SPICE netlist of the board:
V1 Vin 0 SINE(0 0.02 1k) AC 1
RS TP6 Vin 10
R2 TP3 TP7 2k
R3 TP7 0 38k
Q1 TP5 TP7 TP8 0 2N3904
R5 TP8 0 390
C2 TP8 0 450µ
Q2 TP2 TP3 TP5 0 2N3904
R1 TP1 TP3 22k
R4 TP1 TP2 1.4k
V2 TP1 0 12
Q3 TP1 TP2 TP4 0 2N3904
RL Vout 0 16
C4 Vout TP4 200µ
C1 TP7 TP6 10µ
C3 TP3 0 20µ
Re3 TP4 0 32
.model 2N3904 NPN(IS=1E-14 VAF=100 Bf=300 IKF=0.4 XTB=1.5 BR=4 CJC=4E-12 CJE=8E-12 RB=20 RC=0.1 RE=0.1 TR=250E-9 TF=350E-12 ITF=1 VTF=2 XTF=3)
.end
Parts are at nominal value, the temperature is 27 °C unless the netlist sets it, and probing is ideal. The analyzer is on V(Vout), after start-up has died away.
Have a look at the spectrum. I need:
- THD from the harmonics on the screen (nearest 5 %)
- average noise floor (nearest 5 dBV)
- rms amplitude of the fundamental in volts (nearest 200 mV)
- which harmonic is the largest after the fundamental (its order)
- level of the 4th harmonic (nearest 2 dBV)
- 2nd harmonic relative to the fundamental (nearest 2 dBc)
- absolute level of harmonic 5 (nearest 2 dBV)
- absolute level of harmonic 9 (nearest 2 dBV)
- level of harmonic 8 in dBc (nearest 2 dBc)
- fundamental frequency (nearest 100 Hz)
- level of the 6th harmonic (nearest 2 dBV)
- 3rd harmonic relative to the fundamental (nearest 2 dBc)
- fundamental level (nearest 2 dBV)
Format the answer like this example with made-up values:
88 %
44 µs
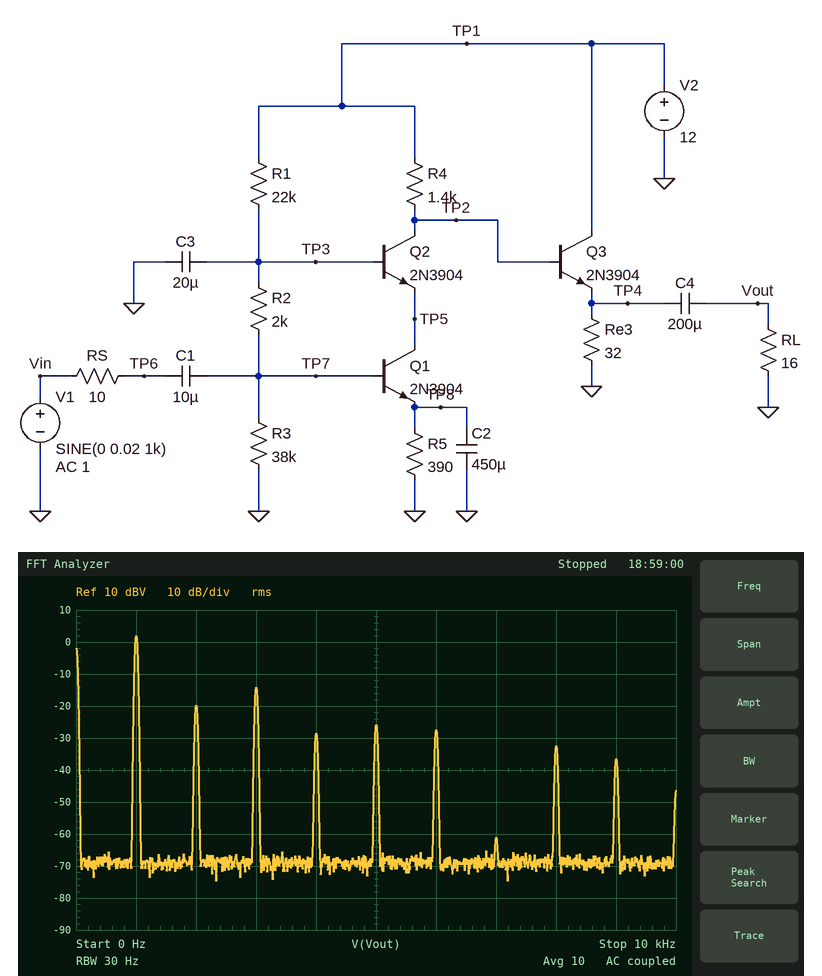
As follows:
20 %
-70 dBV
1.2 V
3
-28 dBV
-22 dBc
-26 dBV
-36 dBV
-34 dBc
1.0 kHz
-28 dBV
-16 dBc
2 dBV
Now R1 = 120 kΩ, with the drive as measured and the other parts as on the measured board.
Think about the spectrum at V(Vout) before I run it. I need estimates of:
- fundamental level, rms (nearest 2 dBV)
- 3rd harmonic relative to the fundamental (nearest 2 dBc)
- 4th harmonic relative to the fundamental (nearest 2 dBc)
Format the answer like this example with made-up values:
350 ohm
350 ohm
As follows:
2 dBV
-28 dBc
-26 dBc
